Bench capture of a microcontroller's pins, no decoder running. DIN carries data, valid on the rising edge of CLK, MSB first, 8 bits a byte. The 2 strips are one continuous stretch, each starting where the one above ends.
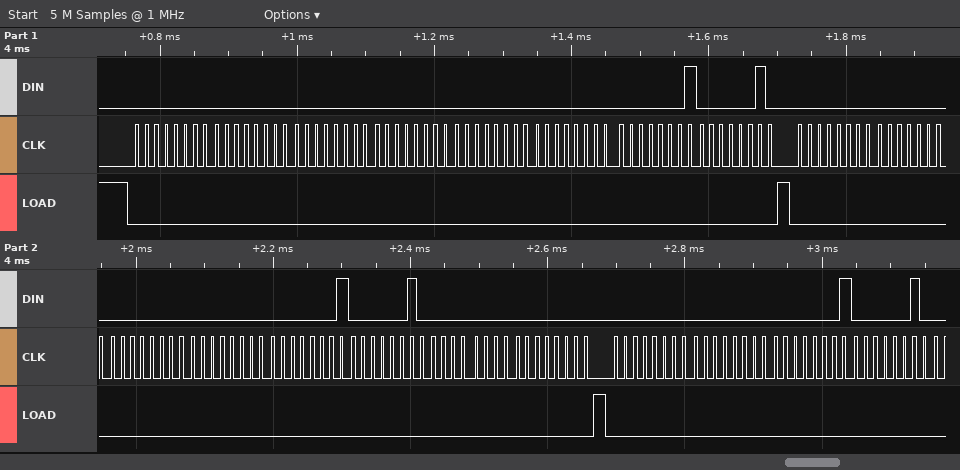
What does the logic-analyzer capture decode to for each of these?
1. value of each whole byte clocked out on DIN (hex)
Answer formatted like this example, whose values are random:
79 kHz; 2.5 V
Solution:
00 00 00 00 00 00 01 02 00 00 00 00 01 02 00 00 00 00 01 02
